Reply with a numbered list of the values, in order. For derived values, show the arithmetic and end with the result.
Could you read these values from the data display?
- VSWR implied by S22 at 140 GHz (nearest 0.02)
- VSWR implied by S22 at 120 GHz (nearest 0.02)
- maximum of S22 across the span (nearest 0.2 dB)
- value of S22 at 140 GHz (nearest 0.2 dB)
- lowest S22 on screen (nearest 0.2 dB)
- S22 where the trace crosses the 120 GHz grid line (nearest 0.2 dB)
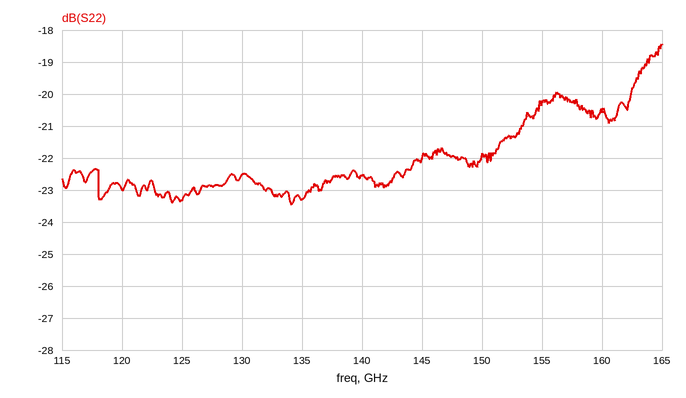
1. |Γ| = 10^(-22.6/20) = 0.0741; VSWR = (1 + 0.0741)/(1 − 0.0741) ≈ 1.16
2. |Γ| = 10^(-23/20) = 0.0708; VSWR = (1 + 0.0708)/(1 − 0.0708) ≈ 1.15, so 1.16 to the nearest 0.02
3. -18.4 dB
4. -22.6 dB
5. -23.4 dB
6. -23.0 dB
